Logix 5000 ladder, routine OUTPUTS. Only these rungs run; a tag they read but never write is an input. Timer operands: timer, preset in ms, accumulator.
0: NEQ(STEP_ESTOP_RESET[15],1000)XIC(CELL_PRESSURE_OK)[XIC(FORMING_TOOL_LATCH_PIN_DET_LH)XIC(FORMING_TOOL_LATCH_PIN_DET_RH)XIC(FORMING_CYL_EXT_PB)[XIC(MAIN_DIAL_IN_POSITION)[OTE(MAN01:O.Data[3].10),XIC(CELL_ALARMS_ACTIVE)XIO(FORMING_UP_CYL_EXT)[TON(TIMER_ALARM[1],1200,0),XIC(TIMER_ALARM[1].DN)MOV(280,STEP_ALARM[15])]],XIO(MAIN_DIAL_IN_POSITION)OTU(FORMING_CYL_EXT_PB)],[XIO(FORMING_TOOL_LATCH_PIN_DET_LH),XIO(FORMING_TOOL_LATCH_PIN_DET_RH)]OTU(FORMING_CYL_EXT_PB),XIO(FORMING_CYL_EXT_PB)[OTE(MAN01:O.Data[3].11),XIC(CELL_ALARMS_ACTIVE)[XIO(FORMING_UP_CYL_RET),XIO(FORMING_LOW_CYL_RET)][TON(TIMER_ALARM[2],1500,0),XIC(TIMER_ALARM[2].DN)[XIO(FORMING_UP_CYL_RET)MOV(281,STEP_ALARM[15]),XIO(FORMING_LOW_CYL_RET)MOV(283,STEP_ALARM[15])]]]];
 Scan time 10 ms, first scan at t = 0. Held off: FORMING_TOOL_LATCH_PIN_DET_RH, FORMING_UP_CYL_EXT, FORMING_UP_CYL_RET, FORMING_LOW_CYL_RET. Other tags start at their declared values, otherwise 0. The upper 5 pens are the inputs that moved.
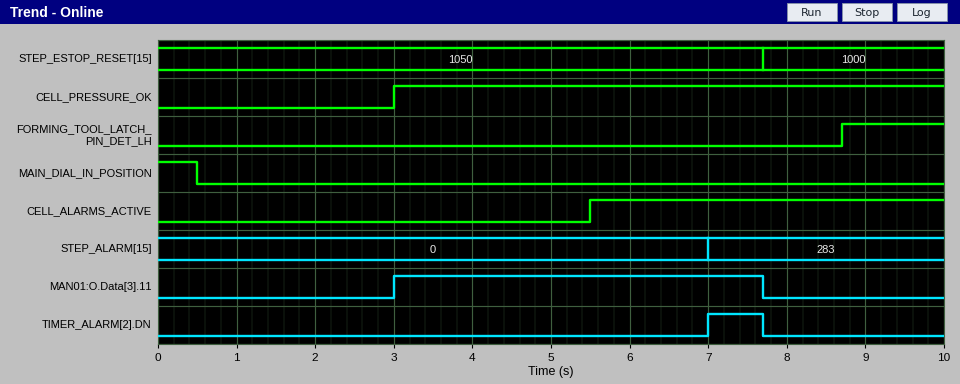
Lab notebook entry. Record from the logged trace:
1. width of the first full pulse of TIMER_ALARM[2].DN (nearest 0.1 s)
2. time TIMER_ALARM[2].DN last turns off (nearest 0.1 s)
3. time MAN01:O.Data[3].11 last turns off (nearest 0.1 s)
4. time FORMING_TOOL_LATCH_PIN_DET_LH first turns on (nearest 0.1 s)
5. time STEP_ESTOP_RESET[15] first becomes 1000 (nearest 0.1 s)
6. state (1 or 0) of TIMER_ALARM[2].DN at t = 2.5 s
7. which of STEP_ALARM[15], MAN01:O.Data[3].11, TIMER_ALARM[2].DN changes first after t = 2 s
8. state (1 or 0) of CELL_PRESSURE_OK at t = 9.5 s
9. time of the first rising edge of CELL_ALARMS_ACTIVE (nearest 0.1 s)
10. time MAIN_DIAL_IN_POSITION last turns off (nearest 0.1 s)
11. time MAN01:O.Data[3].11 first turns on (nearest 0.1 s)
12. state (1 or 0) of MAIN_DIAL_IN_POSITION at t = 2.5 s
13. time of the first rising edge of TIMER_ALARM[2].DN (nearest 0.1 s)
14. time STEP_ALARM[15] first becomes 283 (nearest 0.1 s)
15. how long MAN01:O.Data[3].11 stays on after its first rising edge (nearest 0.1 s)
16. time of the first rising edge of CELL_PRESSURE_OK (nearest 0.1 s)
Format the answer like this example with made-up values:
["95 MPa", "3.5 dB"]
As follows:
["0.7 s", "7.7 s", "7.7 s", "8.7 s", "7.7 s", "0", "MAN01:O.Data[3].11", "1", "5.5 s", "0.5 s", "3.0 s", "0", "7.0 s", "7.0 s", "4.7 s", "3.0 s"]
